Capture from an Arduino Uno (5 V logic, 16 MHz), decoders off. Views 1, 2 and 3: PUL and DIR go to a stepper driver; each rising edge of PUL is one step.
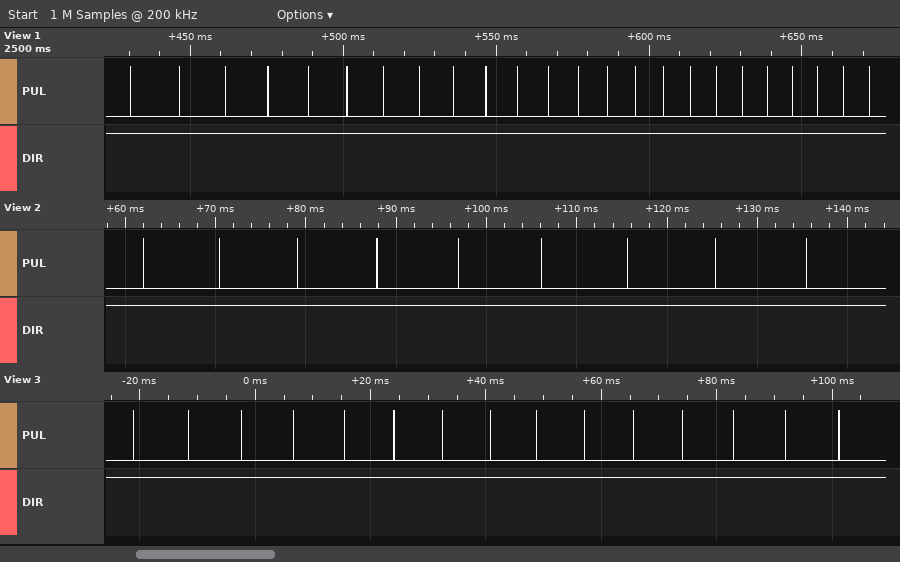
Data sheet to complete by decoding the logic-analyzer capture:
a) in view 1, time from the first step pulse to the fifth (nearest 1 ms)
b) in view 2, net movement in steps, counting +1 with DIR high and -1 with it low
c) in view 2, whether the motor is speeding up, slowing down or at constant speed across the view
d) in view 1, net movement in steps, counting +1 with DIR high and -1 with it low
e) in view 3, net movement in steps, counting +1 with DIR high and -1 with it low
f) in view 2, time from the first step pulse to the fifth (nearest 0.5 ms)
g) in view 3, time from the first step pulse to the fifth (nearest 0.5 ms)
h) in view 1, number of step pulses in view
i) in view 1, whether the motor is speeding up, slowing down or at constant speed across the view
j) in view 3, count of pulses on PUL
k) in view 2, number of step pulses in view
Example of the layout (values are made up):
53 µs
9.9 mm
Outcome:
58 ms
+9
slowing down
+24
+15
35.0 ms
36.5 ms
24
speeding up
15
9
